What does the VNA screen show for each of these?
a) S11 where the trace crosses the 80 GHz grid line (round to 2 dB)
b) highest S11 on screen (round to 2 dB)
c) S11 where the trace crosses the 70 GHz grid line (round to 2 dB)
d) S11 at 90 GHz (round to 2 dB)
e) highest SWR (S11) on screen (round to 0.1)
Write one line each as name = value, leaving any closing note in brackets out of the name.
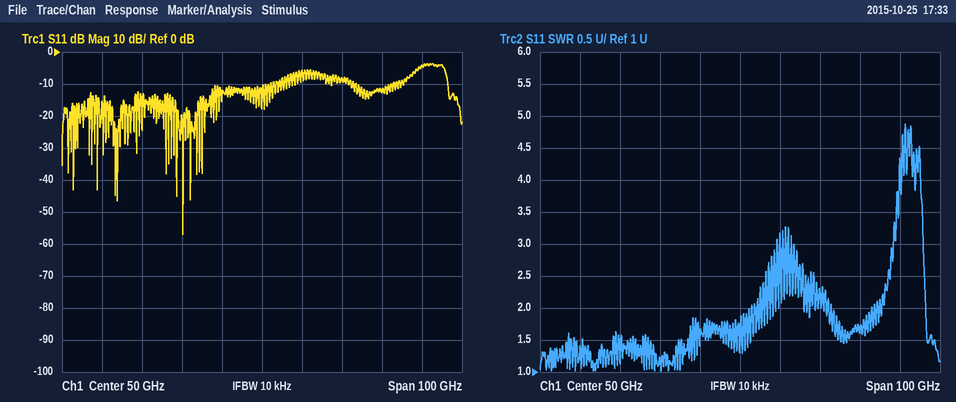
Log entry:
S11 where the trace crosses the 80 GHz grid line = -12 dB
highest S11 on screen = -4 dB
S11 where the trace crosses the 70 GHz grid line = -8 dB
S11 at 90 GHz = -4 dB
highest SWR (S11) on screen = 4.9
